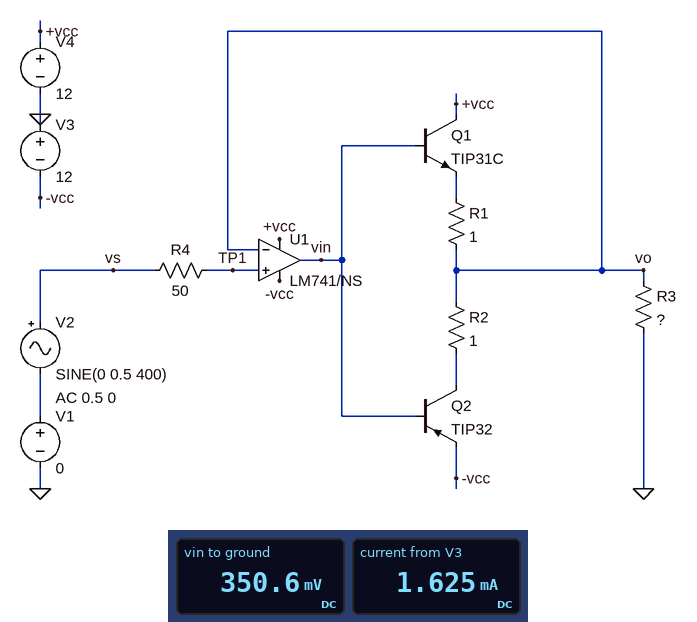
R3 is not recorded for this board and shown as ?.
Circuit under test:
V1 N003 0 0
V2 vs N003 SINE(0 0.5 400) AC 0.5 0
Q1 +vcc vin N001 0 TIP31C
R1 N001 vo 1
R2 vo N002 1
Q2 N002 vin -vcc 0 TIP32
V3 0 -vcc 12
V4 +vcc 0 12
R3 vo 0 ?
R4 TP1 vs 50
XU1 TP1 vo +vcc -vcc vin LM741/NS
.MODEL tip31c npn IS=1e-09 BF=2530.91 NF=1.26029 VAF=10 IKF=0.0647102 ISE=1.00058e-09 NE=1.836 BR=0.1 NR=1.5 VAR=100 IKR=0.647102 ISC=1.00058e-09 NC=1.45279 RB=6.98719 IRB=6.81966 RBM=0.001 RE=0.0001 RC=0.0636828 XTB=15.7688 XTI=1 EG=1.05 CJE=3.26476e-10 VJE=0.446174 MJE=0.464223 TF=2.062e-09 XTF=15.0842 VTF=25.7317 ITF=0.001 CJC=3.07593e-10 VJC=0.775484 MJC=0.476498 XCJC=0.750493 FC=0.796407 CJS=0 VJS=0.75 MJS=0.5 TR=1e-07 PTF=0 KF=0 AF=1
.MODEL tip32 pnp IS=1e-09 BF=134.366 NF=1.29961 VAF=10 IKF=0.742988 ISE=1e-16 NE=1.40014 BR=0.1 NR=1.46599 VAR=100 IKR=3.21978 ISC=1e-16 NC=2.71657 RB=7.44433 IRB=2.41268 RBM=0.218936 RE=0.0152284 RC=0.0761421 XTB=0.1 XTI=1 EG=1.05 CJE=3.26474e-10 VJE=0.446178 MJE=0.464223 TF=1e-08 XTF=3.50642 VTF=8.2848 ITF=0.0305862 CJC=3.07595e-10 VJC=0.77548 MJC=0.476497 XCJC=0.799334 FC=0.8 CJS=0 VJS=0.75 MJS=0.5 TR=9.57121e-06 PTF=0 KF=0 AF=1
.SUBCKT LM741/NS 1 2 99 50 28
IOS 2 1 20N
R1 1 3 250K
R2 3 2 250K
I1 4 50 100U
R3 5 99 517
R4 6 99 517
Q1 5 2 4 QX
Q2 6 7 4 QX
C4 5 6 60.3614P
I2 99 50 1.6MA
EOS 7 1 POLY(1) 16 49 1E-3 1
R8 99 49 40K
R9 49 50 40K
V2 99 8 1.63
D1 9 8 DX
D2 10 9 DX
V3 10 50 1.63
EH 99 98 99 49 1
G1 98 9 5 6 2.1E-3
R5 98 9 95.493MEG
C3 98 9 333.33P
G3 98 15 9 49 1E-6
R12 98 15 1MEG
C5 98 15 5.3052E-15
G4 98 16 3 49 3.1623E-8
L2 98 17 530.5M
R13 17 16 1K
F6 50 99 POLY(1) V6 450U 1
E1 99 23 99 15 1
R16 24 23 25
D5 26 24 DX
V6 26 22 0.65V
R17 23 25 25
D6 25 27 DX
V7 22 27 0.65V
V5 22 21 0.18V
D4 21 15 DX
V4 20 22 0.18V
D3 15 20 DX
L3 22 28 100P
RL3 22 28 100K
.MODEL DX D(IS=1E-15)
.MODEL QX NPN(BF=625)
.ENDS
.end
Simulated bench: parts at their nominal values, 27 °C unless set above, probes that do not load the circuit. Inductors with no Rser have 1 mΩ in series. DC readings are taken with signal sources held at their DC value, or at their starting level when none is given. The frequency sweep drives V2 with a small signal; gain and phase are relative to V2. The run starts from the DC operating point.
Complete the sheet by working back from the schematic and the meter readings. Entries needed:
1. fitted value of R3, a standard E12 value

10 Ω
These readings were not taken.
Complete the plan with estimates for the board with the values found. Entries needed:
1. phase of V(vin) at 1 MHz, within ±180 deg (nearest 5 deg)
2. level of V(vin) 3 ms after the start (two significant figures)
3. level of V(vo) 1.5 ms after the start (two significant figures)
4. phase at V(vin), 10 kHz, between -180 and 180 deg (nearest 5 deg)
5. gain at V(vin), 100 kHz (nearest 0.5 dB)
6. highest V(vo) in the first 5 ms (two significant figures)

-155 deg
1.1 V
-270 mV
-20 deg
19.5 dB
500 mV
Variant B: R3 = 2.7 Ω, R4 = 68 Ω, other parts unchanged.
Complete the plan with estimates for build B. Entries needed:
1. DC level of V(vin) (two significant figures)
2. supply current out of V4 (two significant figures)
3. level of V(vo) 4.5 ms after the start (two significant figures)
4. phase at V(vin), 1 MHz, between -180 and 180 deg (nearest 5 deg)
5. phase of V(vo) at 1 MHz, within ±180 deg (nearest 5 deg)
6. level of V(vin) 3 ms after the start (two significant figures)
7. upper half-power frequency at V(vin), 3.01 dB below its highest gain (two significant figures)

390 mV
2.0 mA
-75 mV
-160 deg
-135 deg
1.3 V
30 kHz
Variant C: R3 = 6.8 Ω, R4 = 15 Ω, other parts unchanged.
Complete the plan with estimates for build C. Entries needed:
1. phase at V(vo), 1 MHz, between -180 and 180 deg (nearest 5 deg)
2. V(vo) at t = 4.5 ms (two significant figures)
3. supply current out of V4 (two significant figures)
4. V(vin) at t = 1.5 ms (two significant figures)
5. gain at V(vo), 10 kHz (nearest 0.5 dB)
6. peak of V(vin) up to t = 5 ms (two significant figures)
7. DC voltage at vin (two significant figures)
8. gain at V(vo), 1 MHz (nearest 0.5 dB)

-110 deg
-190 mV
1.8 mA
-960 mV
-0.5 dB
1.2 V
360 mV
-31.0 dB
